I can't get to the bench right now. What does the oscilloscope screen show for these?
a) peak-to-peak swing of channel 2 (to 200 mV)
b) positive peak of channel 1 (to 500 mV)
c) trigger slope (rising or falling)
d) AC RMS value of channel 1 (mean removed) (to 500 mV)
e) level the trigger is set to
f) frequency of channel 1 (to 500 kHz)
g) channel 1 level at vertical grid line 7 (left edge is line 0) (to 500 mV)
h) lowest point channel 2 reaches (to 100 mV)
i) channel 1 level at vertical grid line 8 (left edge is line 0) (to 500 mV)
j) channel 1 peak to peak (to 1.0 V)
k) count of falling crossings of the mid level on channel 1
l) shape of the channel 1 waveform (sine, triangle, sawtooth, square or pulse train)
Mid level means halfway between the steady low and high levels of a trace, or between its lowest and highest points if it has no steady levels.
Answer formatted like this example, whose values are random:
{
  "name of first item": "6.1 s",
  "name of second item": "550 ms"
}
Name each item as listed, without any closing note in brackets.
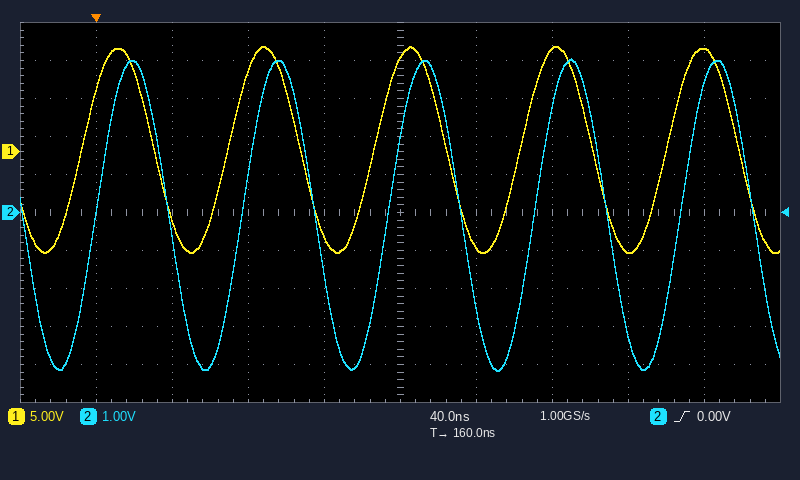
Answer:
{
  "peak-to-peak swing of channel 2": "8.2 V",
  "positive peak of channel 1": "14.0 V",
  "trigger slope": "rising",
  "AC RMS value of channel 1 (mean removed)": "9.5 V",
  "level the trigger is set to": "0.00 V",
  "frequency of channel 1": "13.0 MHz",
  "channel 1 level at vertical grid line 7 (left edge is line 0)": "13.5 V",
  "lowest point channel 2 reaches": "-4.2 V",
  "channel 1 level at vertical grid line 8 (left edge is line 0)": "-13.0 V",
  "channel 1 peak to peak": "27.0 V",
  "count of falling crossings of the mid level on channel 1": "5",
  "shape of the channel 1 waveform": "sine"
}
